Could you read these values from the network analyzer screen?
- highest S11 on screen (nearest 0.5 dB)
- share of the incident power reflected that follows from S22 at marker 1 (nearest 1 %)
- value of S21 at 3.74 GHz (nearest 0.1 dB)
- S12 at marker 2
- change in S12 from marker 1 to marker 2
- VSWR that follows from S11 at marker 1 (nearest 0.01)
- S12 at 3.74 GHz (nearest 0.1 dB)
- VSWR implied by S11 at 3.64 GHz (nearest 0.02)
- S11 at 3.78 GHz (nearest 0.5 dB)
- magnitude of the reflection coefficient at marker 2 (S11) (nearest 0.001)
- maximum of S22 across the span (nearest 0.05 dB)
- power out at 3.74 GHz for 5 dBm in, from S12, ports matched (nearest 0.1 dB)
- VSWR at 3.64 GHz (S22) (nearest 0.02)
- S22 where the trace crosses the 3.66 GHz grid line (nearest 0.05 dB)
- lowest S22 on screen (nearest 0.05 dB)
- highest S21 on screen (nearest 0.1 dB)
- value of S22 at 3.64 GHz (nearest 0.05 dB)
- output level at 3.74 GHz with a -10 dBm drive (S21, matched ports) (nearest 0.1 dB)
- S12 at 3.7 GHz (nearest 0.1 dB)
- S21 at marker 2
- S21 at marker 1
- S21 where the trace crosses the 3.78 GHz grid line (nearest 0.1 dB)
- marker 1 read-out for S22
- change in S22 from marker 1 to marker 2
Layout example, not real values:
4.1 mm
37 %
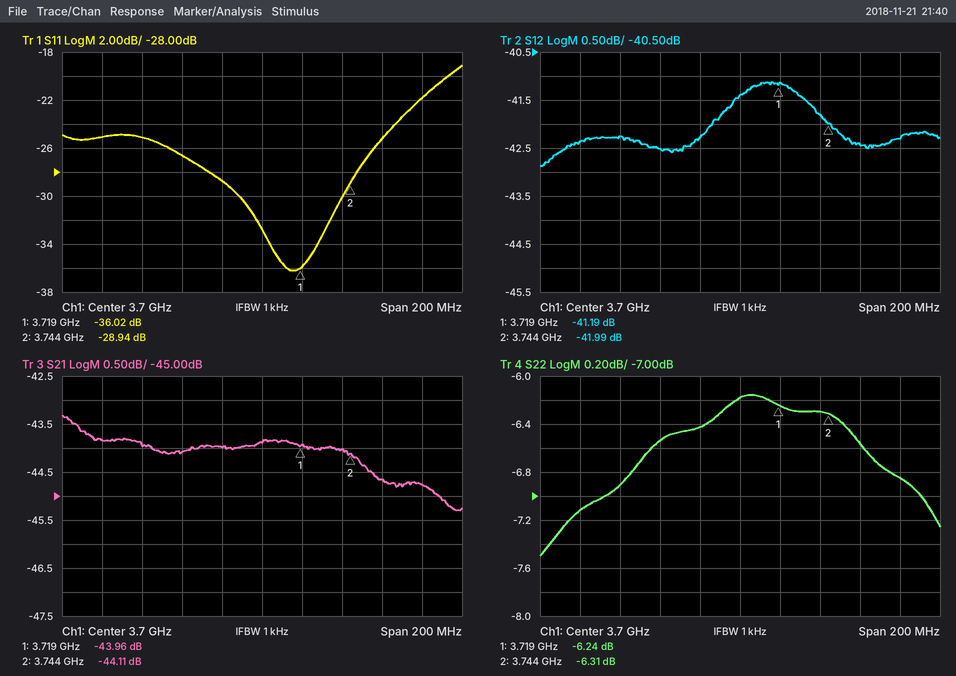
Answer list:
-19.0 dB
24 %
-44.0 dB
-41.99 dB
-0.80 dB
1.03
-41.8 dB
1.12
-22.0 dB
0.036
-6.15 dB
-36.8 dBm
2.64
-6.55 dB
-7.50 dB
-43.3 dB
-6.90 dB
-54.0 dBm
-41.4 dB
-44.11 dB
-43.96 dB
-44.8 dB
-6.24 dB
-0.07 dB
